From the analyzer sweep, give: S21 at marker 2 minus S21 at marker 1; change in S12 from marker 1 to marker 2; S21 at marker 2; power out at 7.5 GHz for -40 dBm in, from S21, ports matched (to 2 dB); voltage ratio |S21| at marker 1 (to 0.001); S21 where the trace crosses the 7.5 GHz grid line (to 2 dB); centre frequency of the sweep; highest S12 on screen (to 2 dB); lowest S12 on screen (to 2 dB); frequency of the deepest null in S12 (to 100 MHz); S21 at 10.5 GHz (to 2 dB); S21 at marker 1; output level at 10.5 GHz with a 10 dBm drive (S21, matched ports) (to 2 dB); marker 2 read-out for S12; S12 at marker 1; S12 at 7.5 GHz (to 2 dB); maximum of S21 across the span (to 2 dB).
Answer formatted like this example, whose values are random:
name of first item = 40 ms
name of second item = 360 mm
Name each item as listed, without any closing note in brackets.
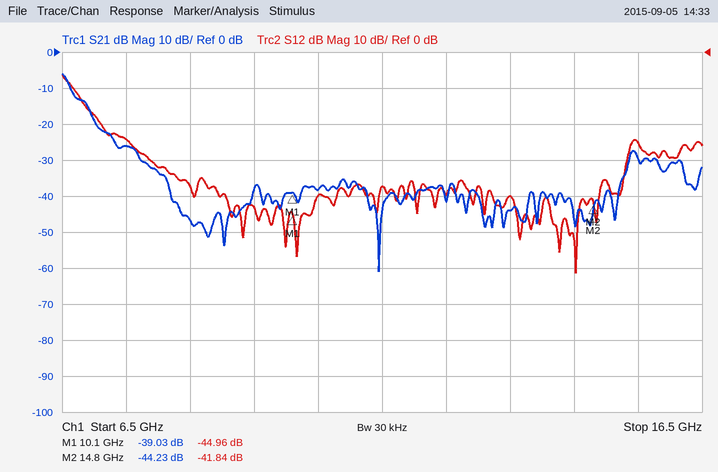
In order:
S21 at marker 2 minus S21 at marker 1 = -5.20 dB
change in S12 from marker 1 to marker 2 = 3.12 dB
S21 at marker 2 = -44.23 dB
power out at 7.5 GHz for -40 dBm in, from S21, ports matched = -66 dBm
voltage ratio |S21| at marker 1 = 0.011
S21 where the trace crosses the 7.5 GHz grid line = -26 dB
centre frequency of the sweep = 11.5 GHz
highest S12 on screen = -6 dB
lowest S12 on screen = -62 dB
frequency of the deepest null in S12 = 14.5 GHz
S21 at 10.5 GHz = -38 dB
S21 at marker 1 = -39.03 dB
output level at 10.5 GHz with a 10 dBm drive (S21, matched ports) = -28 dBm
marker 2 read-out for S12 = -41.84 dB
S12 at marker 1 = -44.96 dB
S12 at 7.5 GHz = -24 dB
maximum of S21 across the span = -6 dB
